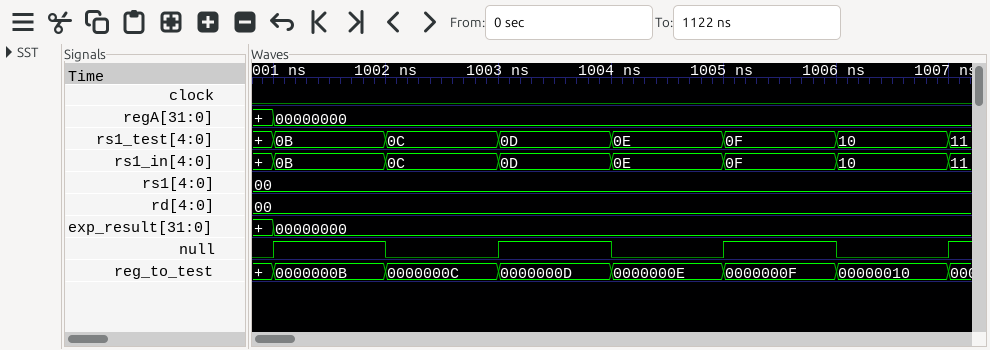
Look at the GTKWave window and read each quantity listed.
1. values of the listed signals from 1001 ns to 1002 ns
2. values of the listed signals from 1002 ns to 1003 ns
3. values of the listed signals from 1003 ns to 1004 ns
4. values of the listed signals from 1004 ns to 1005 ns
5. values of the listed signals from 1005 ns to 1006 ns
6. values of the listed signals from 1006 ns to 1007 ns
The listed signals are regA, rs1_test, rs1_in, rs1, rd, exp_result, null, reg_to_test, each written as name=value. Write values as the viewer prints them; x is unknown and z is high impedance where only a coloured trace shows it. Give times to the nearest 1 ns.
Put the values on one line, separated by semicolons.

regA=00000000, rs1_test=0B, rs1_in=0B, rs1=00, rd=00, exp_result=00000000, null=1, reg_to_test=0000000B; regA=00000000, rs1_test=0C, rs1_in=0C, rs1=00, rd=00, exp_result=00000000, null=0, reg_to_test=0000000C; regA=00000000, rs1_test=0D, rs1_in=0D, rs1=00, rd=00, exp_result=00000000, null=1, reg_to_test=0000000D; regA=00000000, rs1_test=0E, rs1_in=0E, rs1=00, rd=00, exp_result=00000000, null=0, reg_to_test=0000000E; regA=00000000, rs1_test=0F, rs1_in=0F, rs1=00, rd=00, exp_result=00000000, null=1, reg_to_test=0000000F; regA=00000000, rs1_test=10, rs1_in=10, rs1=00, rd=00, exp_result=00000000, null=0, reg_to_test=00000010
